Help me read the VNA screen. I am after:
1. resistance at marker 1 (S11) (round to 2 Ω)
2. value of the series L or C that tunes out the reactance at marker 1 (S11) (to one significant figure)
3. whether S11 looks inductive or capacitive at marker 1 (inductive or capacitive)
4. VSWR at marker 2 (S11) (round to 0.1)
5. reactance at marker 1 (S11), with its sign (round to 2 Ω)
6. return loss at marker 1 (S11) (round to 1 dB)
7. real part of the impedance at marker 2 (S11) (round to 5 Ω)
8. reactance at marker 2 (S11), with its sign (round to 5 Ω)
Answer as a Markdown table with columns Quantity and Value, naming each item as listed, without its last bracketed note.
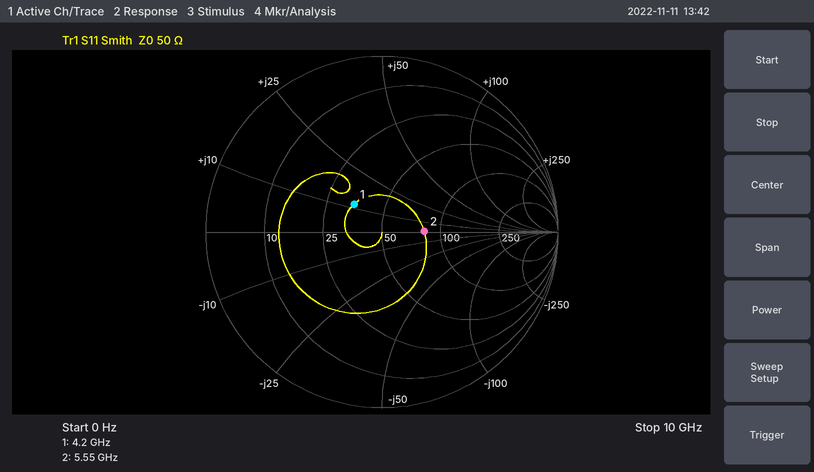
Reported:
| Quantity | Value |
|---|---|
| resistance at marker 1 (S11) | 34 Ω |
| value of the series L or C that tunes out the reactance at marker 1 (S11) | 3 pF |
| whether S11 looks inductive or capacitive at marker 1 | inductive |
| VSWR at marker 2 (S11) | 1.6 |
| reactance at marker 1 (S11), with its sign | +12 Ω |
| return loss at marker 1 (S11) | 13 dB |
| real part of the impedance at marker 2 (S11) | 80 Ω |
| reactance at marker 2 (S11), with its sign | 0 Ω |
